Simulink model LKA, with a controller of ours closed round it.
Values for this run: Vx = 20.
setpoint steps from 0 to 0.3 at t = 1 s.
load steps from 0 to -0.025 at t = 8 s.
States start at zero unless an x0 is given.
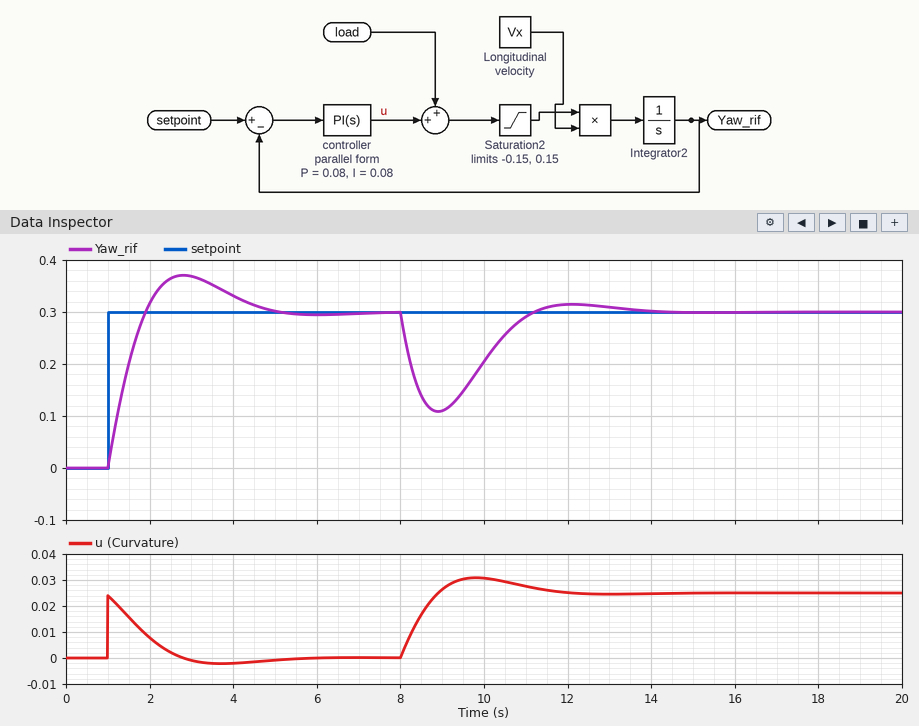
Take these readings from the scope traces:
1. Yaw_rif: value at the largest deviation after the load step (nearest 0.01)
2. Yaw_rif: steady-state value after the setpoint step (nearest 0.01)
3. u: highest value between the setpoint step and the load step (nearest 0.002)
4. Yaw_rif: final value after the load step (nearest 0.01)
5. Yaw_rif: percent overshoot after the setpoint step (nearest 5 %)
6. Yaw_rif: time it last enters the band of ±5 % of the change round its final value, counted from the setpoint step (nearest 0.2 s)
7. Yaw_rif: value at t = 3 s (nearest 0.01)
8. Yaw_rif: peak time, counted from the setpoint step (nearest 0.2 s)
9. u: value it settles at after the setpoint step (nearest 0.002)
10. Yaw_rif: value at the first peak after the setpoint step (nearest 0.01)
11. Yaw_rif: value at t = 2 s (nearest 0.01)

0.11
0.30
0.024
0.30
25 %
3.4 s
0.37
1.8 s
0.000
0.37
0.32
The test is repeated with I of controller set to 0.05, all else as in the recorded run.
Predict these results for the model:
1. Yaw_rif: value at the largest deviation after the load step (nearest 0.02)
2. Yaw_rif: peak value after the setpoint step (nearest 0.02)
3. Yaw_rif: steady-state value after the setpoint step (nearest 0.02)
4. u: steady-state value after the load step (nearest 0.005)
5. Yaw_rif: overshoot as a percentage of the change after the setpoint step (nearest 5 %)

0.08
0.36
0.30
0.025
20 %
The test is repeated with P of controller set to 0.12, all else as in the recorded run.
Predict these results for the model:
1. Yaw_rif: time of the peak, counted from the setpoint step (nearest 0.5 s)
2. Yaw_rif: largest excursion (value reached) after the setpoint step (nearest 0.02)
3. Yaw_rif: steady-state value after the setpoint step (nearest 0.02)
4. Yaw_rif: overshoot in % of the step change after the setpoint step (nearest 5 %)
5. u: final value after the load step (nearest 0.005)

1.5 s
0.34
0.30
15 %
0.025
